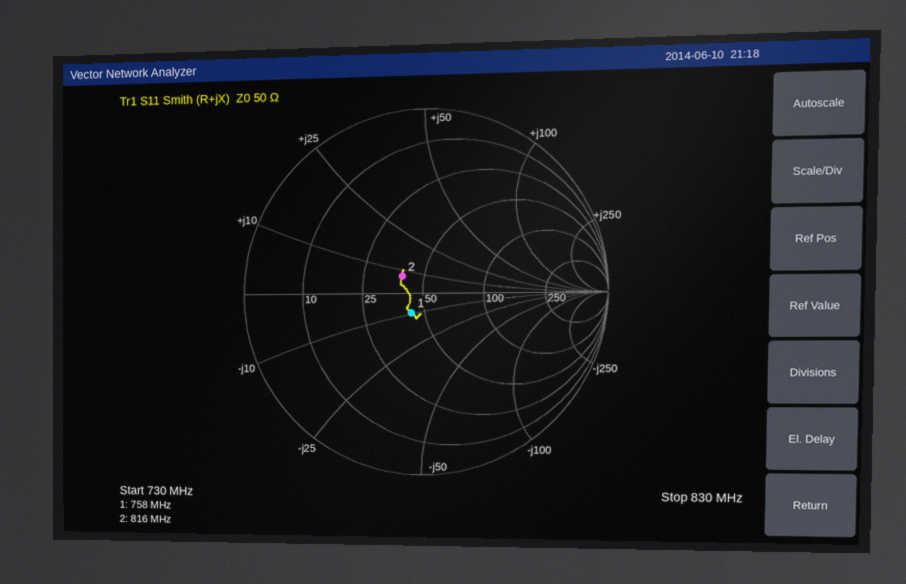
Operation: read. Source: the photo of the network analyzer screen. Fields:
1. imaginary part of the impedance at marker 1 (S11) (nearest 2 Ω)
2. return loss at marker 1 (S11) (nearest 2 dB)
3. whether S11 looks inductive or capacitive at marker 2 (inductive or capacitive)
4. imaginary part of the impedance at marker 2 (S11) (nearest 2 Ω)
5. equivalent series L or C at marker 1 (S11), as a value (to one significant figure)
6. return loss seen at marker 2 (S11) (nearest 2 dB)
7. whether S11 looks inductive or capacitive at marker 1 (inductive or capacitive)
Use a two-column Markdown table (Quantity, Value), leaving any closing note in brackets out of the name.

| Quantity | Value |
|---|---|
| imaginary part of the impedance at marker 1 (S11) | -10 Ω |
| return loss at marker 1 (S11) | 18 dB |
| whether S11 looks inductive or capacitive at marker 2 | inductive |
| imaginary part of the impedance at marker 2 (S11) | +8 Ω |
| equivalent series L or C at marker 1 (S11), as a value | 20 pF |
| return loss seen at marker 2 (S11) | 16 dB |
| whether S11 looks inductive or capacitive at marker 1 | capacitive |
